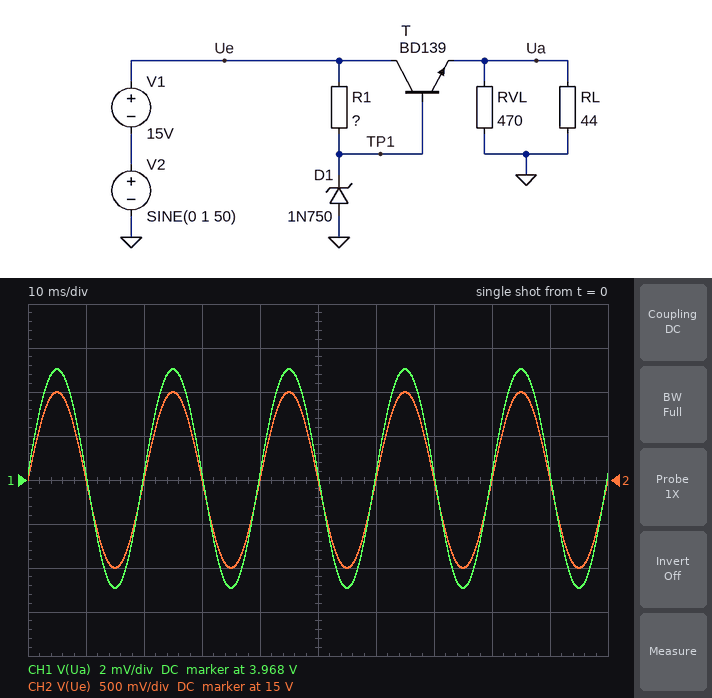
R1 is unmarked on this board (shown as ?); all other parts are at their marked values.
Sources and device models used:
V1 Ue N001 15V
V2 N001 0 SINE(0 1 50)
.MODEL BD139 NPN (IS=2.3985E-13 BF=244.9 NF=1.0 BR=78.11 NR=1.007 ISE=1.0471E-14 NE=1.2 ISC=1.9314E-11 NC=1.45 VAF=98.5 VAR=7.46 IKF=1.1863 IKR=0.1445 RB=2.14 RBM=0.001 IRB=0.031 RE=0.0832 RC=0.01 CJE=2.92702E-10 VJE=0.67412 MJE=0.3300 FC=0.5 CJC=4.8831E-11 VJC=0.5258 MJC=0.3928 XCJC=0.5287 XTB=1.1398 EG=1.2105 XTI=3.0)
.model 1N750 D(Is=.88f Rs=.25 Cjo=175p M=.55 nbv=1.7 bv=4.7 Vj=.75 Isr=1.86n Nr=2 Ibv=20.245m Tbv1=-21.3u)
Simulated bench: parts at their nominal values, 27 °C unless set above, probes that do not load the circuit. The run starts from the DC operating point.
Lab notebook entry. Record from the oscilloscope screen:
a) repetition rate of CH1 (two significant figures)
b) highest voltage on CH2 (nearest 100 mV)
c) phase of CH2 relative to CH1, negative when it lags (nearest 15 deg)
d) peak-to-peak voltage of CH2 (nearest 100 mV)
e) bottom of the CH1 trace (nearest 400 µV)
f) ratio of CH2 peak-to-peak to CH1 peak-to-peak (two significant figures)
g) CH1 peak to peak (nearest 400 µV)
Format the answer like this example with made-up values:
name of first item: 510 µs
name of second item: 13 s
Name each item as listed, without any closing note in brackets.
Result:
repetition rate of CH1: 50 Hz
highest voltage on CH2: 16.0 V
phase of CH2 relative to CH1, negative when it lags: 0 deg
peak-to-peak voltage of CH2: 2.0 V
bottom of the CH1 trace: 3.9632 V
ratio of CH2 peak-to-peak to CH1 peak-to-peak: 200
CH1 peak to peak: 10.0 mV
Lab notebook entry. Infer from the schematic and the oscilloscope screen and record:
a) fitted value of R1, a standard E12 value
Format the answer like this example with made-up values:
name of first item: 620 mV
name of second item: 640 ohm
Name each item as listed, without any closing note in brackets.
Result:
fitted value of R1, a standard E12 value: 1 kΩ
